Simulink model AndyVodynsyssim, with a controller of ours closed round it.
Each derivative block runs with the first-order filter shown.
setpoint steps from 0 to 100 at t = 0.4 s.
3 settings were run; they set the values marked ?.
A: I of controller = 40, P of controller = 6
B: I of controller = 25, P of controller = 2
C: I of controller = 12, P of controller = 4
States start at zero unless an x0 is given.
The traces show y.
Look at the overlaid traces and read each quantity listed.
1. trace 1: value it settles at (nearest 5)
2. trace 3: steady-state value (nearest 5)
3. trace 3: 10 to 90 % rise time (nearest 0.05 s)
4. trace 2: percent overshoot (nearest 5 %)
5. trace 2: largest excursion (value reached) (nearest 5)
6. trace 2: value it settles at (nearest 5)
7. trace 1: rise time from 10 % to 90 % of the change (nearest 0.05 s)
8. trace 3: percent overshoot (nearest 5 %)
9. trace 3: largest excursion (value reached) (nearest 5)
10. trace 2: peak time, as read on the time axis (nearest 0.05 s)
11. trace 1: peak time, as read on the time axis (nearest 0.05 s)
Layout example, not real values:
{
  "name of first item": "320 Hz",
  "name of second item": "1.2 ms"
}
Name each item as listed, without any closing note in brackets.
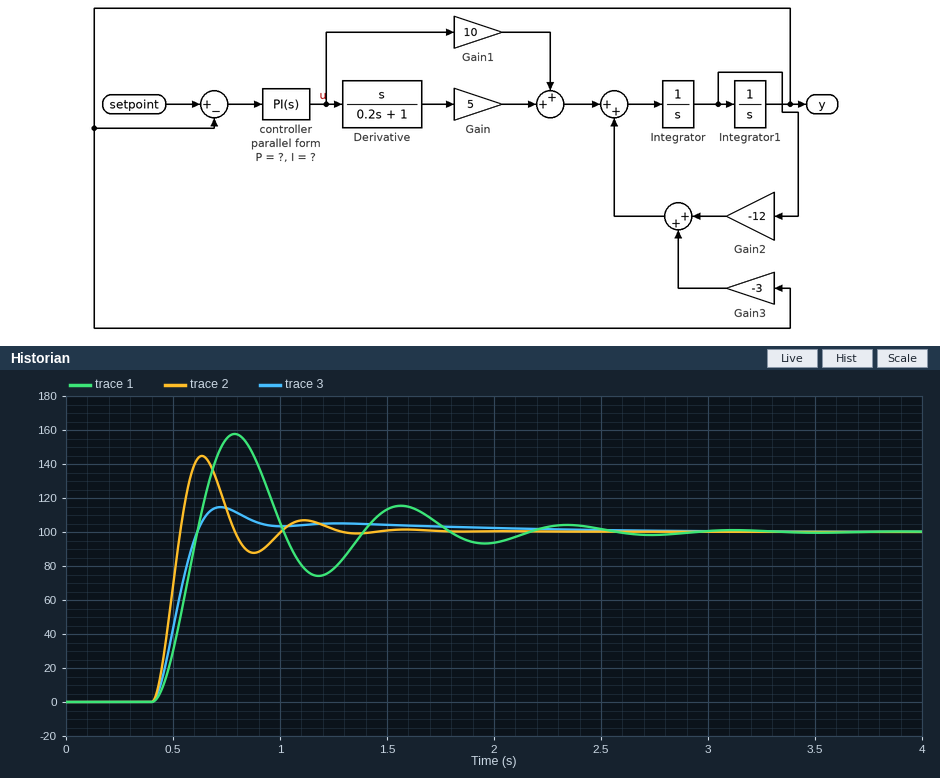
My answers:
{
  "trace 1: value it settles at": "100",
  "trace 3: steady-state value": "100",
  "trace 3: 10 to 90 % rise time": "0.15 s",
  "trace 2: percent overshoot": "45 %",
  "trace 2: largest excursion (value reached)": "145",
  "trace 2: value it settles at": "100",
  "trace 1: rise time from 10 % to 90 % of the change": "0.15 s",
  "trace 3: percent overshoot": "15 %",
  "trace 3: largest excursion (value reached)": "115",
  "trace 2: peak time, as read on the time axis": "0.65 s",
  "trace 1: peak time, as read on the time axis": "0.80 s"
}
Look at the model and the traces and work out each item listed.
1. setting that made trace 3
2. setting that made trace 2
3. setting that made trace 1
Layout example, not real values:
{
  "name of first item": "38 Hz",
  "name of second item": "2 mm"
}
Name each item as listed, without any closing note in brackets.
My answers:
{
  "setting that made trace 3": "C",
  "setting that made trace 2": "A",
  "setting that made trace 1": "B"
}
